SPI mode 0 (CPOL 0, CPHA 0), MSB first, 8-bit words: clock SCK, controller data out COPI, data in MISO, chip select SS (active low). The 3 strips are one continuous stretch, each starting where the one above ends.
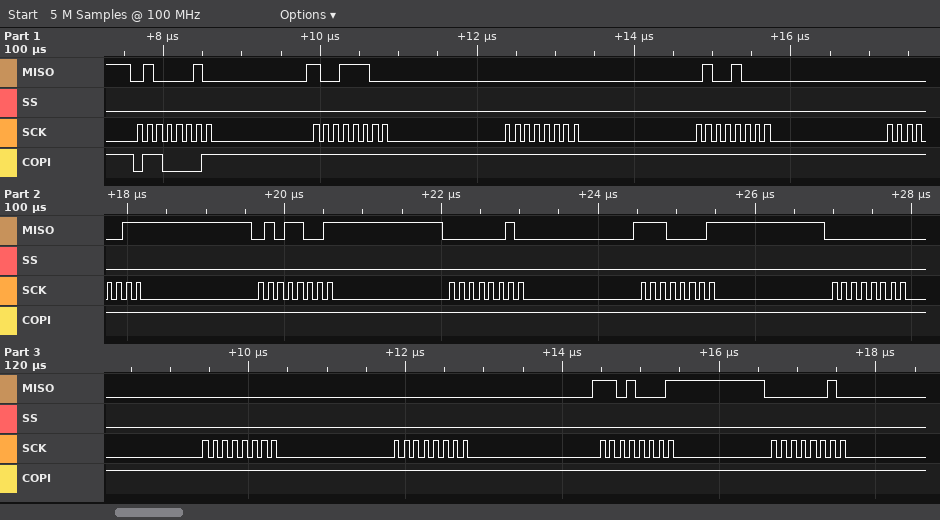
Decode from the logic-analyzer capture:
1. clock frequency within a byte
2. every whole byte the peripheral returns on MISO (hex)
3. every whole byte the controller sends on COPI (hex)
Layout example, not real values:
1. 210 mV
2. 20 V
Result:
1. 8 MHz
2. 42 9C 00 48 03 59 02 E1 00 00 00 D1 02
3. 61 FF FF FF FF FF FF FF FF FF FF FF FF
